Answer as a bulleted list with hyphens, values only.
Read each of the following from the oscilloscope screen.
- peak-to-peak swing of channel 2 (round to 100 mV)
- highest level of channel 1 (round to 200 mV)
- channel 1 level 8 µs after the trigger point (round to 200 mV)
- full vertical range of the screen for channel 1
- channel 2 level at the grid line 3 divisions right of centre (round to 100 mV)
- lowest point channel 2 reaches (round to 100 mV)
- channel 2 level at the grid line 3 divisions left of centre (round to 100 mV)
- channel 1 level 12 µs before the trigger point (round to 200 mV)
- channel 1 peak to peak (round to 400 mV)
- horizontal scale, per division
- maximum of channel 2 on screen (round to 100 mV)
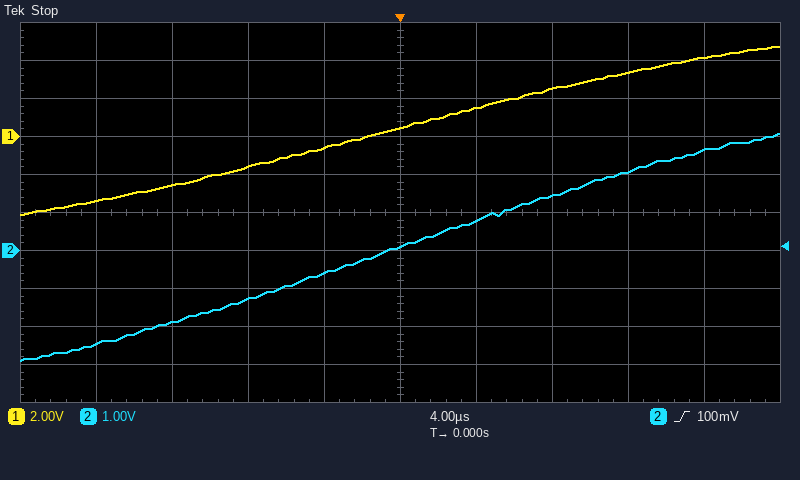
- 6.0 V
- 4.8 V
- 2.6 V
- 20 V
- 2.1 V
- -2.9 V
- -1.9 V
- -2.6 V
- 8.8 V
- 4 µs
- 3.1 V
